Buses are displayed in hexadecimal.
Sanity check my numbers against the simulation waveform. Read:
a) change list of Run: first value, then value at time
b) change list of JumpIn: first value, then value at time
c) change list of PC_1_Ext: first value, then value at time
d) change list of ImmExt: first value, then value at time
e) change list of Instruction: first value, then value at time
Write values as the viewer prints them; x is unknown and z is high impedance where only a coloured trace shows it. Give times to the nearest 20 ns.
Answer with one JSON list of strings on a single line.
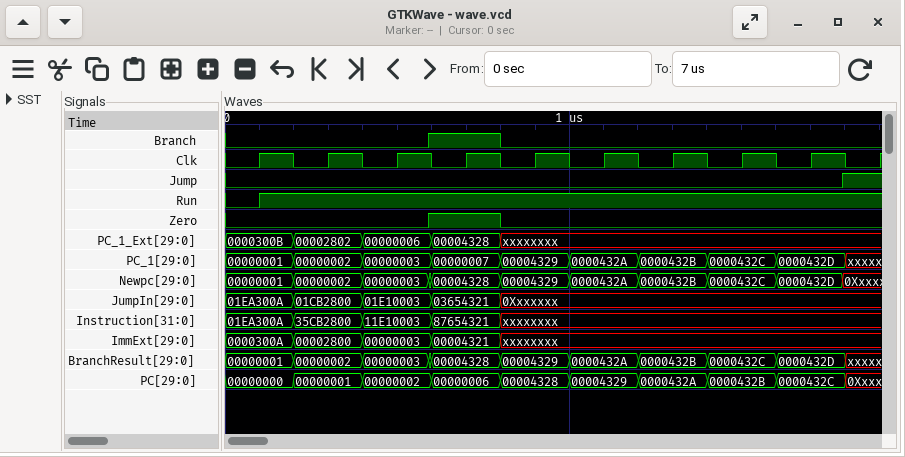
["0, 1 at 100 ns", "01EA300A, 01CB2800 at 200 ns, 01E10003 at 400 ns, 03654321 at 600 ns, 0Xxxxxxx at 800 ns", "0000300B, 00002802 at 200 ns, 00000006 at 400 ns, 00004328 at 600 ns, xxxxxxxx at 800 ns", "0000300A, 00002800 at 200 ns, 00000003 at 400 ns, 00004321 at 600 ns, xxxxxxxx at 800 ns", "01EA300A, 35CB2800 at 200 ns, 11E10003 at 400 ns, 87654321 at 600 ns, xxxxxxxx at 800 ns"]
